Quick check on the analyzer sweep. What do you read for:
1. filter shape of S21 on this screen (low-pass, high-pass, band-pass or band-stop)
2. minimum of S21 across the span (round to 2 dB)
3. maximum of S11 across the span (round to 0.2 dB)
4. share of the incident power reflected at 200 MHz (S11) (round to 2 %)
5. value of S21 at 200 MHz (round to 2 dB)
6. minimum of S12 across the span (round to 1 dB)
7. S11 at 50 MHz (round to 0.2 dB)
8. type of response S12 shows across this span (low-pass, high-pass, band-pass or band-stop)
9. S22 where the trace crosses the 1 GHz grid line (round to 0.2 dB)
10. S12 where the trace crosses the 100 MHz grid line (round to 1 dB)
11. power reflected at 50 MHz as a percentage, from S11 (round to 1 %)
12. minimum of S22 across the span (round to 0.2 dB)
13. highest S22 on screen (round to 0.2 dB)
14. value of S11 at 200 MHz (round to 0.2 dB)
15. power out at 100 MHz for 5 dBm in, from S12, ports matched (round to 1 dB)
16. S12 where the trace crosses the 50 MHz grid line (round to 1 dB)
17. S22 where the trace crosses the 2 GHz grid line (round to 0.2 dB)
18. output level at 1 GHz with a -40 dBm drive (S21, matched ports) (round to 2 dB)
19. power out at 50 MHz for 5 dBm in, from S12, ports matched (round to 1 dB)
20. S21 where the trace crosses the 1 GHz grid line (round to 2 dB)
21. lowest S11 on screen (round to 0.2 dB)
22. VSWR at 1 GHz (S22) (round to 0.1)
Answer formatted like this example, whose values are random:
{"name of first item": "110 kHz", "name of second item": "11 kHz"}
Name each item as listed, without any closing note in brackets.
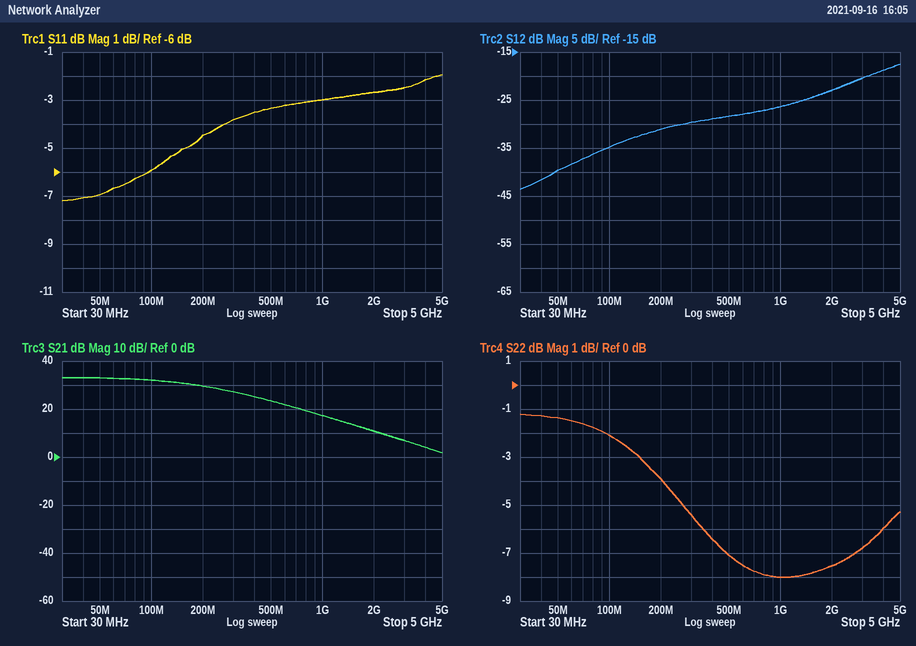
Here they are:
{"filter shape of S21 on this screen": "low-pass", "minimum of S21 across the span": "2 dB", "maximum of S11 across the span": "-2.0 dB", "share of the incident power reflected at 200 MHz (S11)": "36 %", "value of S21 at 200 MHz": "30 dB", "minimum of S12 across the span": "-44 dB", "S11 at 50 MHz": "-7.0 dB", "type of response S12 shows across this span": "high-pass", "S22 where the trace crosses the 1 GHz grid line": "-8.0 dB", "S12 where the trace crosses the 100 MHz grid line": "-35 dB", "power reflected at 50 MHz as a percentage, from S11": "20 %", "minimum of S22 across the span": "-8.0 dB", "highest S22 on screen": "-1.2 dB", "value of S11 at 200 MHz": "-4.4 dB", "power out at 100 MHz for 5 dBm in, from S12, ports matched": "-30 dBm", "S12 where the trace crosses the 50 MHz grid line": "-40 dB", "S22 where the trace crosses the 2 GHz grid line": "-7.6 dB", "output level at 1 GHz with a -40 dBm drive (S21, matched ports)": "-22 dBm", "power out at 50 MHz for 5 dBm in, from S12, ports matched": "-35 dBm", "S21 where the trace crosses the 1 GHz grid line": "18 dB", "lowest S11 on screen": "-7.2 dB", "VSWR at 1 GHz (S22)": "2.3"}
